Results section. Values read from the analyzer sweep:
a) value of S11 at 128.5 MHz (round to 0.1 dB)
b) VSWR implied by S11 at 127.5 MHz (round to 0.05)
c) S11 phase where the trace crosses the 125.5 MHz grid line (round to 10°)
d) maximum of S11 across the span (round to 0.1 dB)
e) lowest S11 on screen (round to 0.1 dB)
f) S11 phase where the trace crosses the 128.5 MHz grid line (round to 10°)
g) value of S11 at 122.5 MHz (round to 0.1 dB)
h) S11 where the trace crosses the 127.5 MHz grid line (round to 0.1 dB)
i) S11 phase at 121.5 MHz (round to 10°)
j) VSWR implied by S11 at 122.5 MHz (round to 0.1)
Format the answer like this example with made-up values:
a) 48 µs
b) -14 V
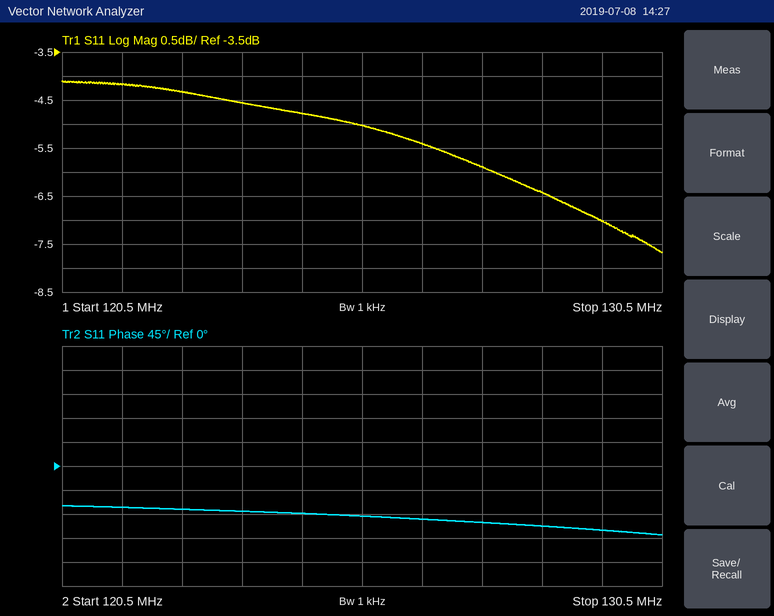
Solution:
a) -6.4 dB
b) 3.05
c) -90°
d) -4.1 dB
e) -7.7 dB
f) -110°
g) -4.3 dB
h) -5.9 dB
i) -80°
j) 4.1
